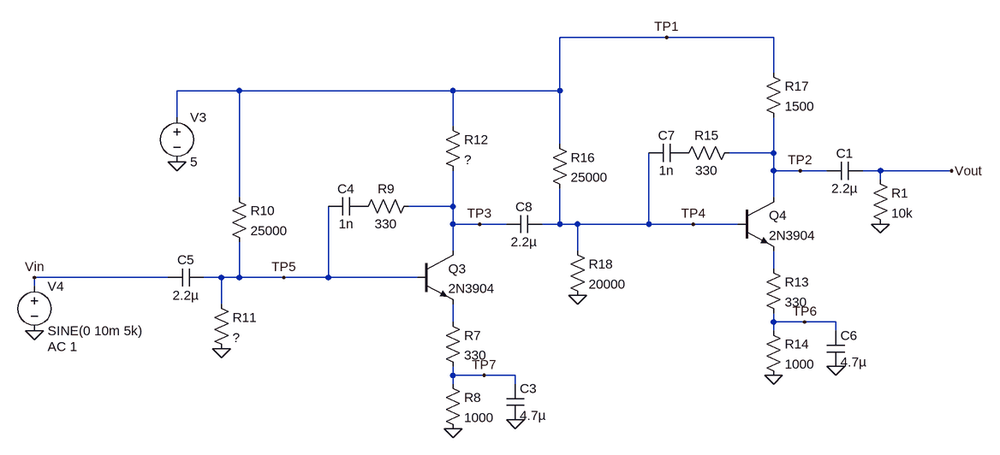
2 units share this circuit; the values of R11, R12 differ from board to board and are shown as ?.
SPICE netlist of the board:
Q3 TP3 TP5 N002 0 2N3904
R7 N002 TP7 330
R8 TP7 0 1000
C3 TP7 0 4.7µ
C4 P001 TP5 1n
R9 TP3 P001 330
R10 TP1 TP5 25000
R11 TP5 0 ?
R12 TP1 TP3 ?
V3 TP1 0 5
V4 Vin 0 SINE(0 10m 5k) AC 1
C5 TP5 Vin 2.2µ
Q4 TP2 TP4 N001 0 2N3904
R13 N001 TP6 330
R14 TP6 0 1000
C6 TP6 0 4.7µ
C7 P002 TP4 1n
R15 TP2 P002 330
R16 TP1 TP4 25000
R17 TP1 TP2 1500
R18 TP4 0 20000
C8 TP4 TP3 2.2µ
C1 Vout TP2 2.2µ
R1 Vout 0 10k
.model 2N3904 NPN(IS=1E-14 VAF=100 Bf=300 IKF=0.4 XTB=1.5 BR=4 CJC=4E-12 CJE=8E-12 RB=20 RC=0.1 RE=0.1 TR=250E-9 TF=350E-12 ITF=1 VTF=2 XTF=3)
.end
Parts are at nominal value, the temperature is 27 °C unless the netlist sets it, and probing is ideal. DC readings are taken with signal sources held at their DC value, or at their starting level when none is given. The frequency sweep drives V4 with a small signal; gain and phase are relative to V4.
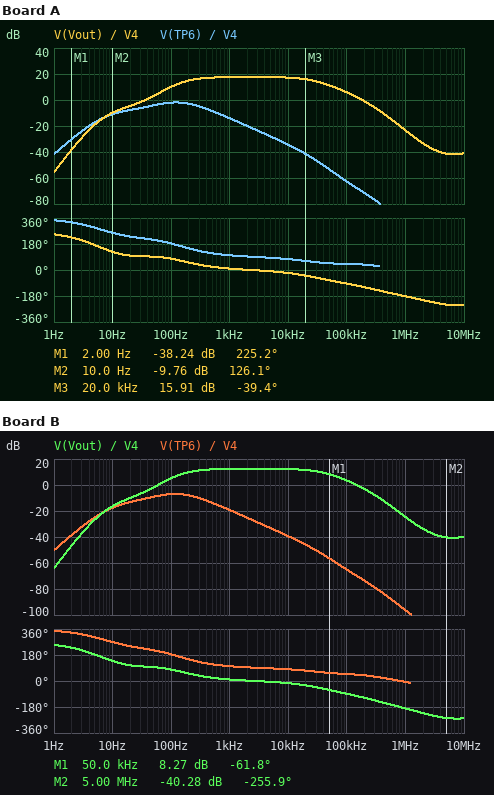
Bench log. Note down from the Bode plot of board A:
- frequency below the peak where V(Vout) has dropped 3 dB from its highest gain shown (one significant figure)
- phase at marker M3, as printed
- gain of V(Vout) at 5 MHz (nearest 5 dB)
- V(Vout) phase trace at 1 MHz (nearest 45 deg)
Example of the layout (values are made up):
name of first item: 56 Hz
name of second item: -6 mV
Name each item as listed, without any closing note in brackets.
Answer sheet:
frequency below the peak where V(Vout) has dropped 3 dB from its highest gain shown: 200 Hz
phase at marker M3, as printed: -39.4 deg
gain of V(Vout) at 5 MHz: -40 dB
V(Vout) phase trace at 1 MHz: -180 deg
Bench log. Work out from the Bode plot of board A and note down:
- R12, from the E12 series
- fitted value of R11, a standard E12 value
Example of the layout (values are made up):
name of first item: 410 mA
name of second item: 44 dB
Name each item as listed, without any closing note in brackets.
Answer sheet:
R12, from the E12 series: 820 Ω
fitted value of R11, a standard E12 value: 15 kΩ
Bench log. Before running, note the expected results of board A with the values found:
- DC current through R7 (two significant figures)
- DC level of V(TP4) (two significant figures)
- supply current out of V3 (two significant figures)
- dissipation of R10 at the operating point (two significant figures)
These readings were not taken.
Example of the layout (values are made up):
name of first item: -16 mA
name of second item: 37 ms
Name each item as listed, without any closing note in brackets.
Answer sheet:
DC current through R7: 900 µA
DC level of V(TP4): 2.2 V
supply current out of V3: 2.3 mA
dissipation of R10 at the operating point: 400 µW
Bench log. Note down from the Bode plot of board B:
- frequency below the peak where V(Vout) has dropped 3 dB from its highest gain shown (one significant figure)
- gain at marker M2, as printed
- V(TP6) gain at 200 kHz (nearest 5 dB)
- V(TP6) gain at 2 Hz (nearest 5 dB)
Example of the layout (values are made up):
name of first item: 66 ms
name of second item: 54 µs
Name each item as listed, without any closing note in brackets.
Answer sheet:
frequency below the peak where V(Vout) has dropped 3 dB from its highest gain shown: 200 Hz
gain at marker M2, as printed: -40.28 dB
V(TP6) gain at 200 kHz: -75 dB
V(TP6) gain at 2 Hz: -40 dB
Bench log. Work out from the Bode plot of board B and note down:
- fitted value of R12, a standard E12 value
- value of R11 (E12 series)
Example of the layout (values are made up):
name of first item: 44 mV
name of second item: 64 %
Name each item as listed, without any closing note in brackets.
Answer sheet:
fitted value of R12, a standard E12 value: 470 Ω
value of R11: 8.2 kΩ
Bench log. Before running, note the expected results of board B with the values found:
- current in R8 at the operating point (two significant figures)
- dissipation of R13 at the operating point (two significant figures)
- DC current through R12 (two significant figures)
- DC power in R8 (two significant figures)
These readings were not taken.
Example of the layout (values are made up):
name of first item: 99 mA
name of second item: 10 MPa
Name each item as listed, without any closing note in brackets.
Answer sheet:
current in R8 at the operating point: 450 µA
dissipation of R13 at the operating point: 430 µW
DC current through R12: 440 µA
DC power in R8: 200 µW
